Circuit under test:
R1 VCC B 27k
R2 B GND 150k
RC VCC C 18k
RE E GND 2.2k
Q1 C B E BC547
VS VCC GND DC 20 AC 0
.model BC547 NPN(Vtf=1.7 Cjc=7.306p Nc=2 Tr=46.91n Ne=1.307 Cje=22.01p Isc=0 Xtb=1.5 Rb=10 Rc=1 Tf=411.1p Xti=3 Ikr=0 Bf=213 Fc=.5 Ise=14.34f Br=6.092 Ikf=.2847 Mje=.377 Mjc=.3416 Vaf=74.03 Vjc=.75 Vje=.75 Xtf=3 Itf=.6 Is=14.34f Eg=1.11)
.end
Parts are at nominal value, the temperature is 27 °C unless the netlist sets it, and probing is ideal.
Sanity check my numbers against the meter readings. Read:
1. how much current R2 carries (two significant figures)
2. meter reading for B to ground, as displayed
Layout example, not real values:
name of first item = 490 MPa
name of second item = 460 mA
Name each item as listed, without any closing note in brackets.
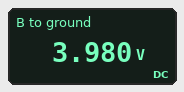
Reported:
how much current R2 carries = 27 µA
meter reading for B to ground, as displayed = 3.980 V
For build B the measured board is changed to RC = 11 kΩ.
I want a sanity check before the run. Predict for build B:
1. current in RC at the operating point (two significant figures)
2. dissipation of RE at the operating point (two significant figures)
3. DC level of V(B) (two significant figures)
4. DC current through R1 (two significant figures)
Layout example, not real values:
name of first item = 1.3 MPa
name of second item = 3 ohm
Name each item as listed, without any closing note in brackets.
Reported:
current in RC at the operating point = 1.4 mA
dissipation of RE at the operating point = 8.4 mW
DC level of V(B) = 5.0 V
DC current through R1 = 560 µA
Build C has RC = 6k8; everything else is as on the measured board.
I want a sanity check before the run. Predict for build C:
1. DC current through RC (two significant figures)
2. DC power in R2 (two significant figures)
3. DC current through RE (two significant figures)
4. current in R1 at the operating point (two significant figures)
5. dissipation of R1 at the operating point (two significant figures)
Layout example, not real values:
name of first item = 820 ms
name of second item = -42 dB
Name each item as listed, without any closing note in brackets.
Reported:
DC current through RC = 2.1 mA
DC power in R2 = 270 µW
DC current through RE = 2.6 mA
current in R1 at the operating point = 510 µA
dissipation of R1 at the operating point = 6.9 mW
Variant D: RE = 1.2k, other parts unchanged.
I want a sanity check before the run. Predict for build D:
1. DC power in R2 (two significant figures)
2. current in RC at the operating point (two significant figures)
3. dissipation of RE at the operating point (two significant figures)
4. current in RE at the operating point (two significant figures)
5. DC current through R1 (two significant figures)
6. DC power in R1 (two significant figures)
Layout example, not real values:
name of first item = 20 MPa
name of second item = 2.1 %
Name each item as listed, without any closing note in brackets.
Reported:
DC power in R2 = 47 µW
current in RC at the operating point = 1.0 mA
dissipation of RE at the operating point = 3.2 mW
current in RE at the operating point = 1.6 mA
DC current through R1 = 640 µA
DC power in R1 = 11 mW
